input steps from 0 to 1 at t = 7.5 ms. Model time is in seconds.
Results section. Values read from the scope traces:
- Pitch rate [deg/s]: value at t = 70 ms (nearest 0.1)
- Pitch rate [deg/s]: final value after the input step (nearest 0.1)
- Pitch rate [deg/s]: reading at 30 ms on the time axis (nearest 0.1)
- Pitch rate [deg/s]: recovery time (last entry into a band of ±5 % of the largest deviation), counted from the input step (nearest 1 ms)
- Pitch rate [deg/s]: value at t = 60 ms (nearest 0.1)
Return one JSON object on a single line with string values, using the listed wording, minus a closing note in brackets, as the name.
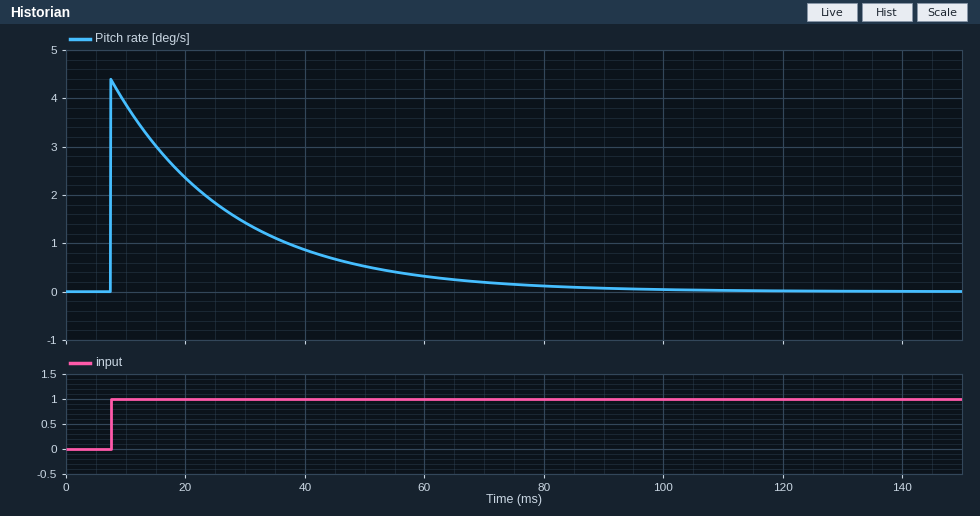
{"Pitch rate [deg/s]: value at t = 70 ms": "0.2", "Pitch rate [deg/s]: final value after the input step": "0.0", "Pitch rate [deg/s]: reading at 30 ms on the time axis": "1.4", "Pitch rate [deg/s]: recovery time (last entry into a band of ±5 % of the largest deviation), counted from the input step": "60 ms", "Pitch rate [deg/s]: value at t = 60 ms": "0.3"}
